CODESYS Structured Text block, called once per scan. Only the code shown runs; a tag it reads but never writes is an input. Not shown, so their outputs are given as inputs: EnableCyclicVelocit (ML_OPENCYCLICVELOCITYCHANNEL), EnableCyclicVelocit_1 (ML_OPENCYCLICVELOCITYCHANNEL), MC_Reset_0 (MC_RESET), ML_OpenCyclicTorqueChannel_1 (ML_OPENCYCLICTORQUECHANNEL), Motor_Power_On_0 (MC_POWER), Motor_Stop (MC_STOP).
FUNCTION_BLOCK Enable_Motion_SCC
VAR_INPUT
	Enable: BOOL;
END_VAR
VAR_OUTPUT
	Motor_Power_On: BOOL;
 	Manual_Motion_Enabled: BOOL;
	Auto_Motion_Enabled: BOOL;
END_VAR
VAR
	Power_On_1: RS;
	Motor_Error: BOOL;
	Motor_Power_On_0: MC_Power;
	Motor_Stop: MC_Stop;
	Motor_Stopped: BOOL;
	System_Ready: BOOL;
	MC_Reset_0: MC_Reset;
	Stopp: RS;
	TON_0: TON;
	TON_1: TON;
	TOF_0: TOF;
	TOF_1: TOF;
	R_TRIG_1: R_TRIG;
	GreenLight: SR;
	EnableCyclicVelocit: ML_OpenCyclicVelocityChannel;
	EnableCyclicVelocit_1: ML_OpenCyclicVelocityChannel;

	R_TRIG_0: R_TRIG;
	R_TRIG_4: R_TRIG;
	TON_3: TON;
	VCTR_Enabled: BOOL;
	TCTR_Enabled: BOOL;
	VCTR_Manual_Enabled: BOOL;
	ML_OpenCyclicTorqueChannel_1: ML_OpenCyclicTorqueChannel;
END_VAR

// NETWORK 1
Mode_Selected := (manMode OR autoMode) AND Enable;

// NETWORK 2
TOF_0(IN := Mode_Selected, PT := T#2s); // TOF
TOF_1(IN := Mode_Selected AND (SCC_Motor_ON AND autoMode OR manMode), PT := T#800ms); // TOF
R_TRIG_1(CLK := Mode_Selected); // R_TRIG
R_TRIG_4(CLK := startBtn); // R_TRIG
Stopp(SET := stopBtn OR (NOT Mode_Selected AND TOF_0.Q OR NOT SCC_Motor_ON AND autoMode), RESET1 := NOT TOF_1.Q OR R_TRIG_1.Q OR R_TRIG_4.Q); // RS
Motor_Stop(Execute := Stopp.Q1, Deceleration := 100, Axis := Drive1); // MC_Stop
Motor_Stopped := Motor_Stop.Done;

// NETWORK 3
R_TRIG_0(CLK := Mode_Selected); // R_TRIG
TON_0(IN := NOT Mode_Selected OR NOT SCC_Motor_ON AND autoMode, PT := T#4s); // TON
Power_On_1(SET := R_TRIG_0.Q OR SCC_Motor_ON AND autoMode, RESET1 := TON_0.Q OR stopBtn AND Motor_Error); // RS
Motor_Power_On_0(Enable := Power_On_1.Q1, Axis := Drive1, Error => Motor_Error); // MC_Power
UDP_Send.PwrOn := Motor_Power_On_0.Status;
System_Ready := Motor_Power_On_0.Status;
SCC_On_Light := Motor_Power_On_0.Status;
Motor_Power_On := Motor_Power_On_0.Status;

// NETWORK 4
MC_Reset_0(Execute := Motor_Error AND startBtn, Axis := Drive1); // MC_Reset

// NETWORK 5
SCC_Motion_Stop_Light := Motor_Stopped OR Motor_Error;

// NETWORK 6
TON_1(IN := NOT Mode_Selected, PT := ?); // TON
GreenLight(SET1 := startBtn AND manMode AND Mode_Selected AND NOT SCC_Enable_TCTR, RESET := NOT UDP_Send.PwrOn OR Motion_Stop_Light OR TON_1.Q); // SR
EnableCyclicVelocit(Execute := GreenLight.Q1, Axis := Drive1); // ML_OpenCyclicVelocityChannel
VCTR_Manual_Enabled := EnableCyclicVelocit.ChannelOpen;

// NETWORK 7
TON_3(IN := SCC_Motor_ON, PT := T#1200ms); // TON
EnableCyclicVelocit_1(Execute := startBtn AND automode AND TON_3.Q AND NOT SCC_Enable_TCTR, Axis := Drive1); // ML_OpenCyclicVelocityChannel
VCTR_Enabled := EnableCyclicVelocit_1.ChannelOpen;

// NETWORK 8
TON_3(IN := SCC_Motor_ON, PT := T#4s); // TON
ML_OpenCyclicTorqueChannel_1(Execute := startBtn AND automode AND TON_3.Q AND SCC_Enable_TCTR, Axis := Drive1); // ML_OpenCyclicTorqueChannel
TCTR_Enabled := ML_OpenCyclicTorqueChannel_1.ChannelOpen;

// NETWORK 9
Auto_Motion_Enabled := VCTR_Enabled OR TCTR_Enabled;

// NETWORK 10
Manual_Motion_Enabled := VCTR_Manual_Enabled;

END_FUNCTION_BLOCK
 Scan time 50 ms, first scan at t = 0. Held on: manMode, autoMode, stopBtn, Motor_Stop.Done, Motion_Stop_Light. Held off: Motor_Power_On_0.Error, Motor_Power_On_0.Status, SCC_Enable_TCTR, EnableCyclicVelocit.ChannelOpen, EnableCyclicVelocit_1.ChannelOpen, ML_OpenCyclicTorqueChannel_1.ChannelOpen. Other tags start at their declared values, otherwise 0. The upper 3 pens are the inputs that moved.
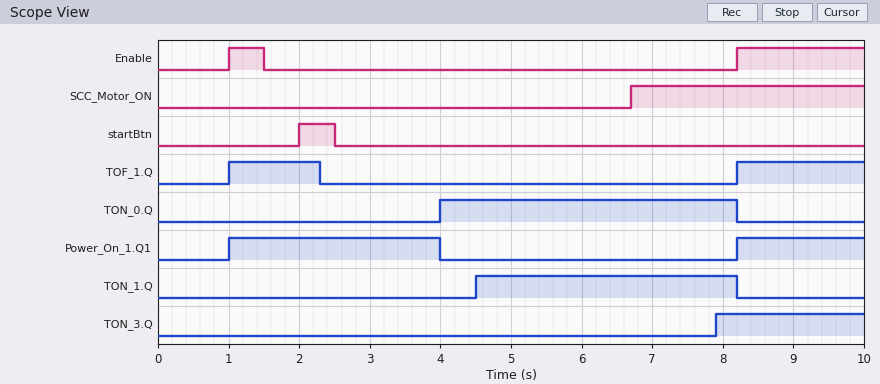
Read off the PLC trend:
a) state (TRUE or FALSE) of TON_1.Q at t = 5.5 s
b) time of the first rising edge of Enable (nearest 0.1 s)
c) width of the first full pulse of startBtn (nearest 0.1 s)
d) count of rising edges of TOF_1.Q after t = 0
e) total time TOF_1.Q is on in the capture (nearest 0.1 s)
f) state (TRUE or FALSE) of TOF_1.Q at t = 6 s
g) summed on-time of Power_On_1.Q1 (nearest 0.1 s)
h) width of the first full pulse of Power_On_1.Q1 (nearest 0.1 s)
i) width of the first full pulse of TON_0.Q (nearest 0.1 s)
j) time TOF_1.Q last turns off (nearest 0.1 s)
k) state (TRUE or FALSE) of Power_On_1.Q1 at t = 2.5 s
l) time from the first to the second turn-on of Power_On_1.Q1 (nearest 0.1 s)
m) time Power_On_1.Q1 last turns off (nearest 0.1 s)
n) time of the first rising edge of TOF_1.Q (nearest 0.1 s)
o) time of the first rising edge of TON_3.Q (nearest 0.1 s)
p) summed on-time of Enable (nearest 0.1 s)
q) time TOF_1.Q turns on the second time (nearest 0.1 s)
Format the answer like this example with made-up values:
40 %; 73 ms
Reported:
TRUE; 1.0 s; 0.5 s; 2; 3.1 s; FALSE; 4.8 s; 3.0 s; 4.2 s; 2.3 s; TRUE; 7.2 s; 4.0 s; 1.0 s; 7.9 s; 2.3 s; 8.2 s
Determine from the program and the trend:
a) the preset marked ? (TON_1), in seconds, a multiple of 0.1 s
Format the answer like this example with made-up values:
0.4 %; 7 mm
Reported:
3.0 s
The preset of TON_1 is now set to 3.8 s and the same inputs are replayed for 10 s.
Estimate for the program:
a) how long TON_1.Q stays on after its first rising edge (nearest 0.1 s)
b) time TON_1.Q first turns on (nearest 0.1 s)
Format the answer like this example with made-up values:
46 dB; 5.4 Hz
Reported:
2.9 s; 5.3 s
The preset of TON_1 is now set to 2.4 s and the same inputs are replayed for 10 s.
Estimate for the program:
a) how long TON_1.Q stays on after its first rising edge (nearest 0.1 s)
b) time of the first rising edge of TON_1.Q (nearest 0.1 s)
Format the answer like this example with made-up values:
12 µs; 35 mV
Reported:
4.3 s; 3.9 s
